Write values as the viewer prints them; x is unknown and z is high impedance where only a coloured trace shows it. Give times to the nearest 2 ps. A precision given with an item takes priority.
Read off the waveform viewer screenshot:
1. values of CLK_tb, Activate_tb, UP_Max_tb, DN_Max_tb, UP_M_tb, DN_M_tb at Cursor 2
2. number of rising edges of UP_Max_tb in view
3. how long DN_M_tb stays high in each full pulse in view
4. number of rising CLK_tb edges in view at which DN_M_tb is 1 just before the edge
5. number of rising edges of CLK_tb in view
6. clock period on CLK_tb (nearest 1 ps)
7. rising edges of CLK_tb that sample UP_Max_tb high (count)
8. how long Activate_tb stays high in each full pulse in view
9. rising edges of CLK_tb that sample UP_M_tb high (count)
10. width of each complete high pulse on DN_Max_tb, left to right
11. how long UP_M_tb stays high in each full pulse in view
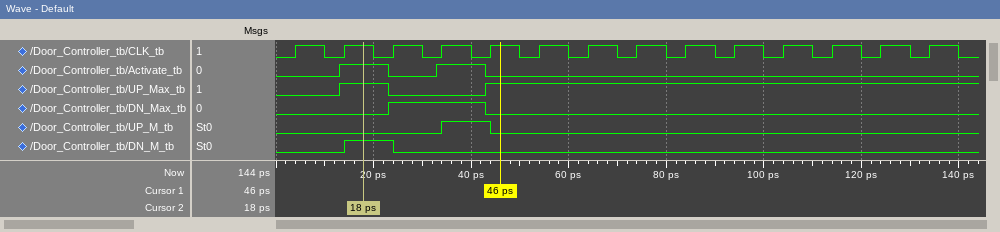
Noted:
CLK_tb=1, Activate_tb=1, UP_Max_tb=1, DN_Max_tb=0, UP_M_tb=0, DN_M_tb=1
2
10 ps
1
14
10 ps
11
10 ps, 10 ps
1
20 ps
10 ps
